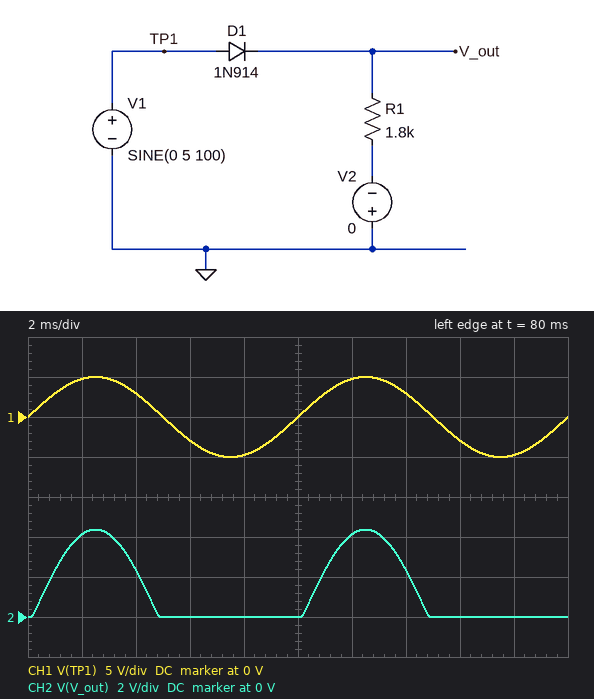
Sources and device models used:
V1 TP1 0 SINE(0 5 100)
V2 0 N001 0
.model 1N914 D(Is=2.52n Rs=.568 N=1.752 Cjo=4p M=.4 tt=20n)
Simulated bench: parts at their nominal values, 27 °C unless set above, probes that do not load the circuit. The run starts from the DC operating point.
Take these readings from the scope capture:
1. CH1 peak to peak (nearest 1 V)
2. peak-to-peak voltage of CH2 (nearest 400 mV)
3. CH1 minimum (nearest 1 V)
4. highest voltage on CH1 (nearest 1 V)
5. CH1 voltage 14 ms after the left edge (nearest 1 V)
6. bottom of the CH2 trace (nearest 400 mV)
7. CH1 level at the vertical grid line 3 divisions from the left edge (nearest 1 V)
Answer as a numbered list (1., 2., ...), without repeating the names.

1. 10 V
2. 4.4 V
3. -5 V
4. 5 V
5. 3 V
6. 0 V
7. -3 V
